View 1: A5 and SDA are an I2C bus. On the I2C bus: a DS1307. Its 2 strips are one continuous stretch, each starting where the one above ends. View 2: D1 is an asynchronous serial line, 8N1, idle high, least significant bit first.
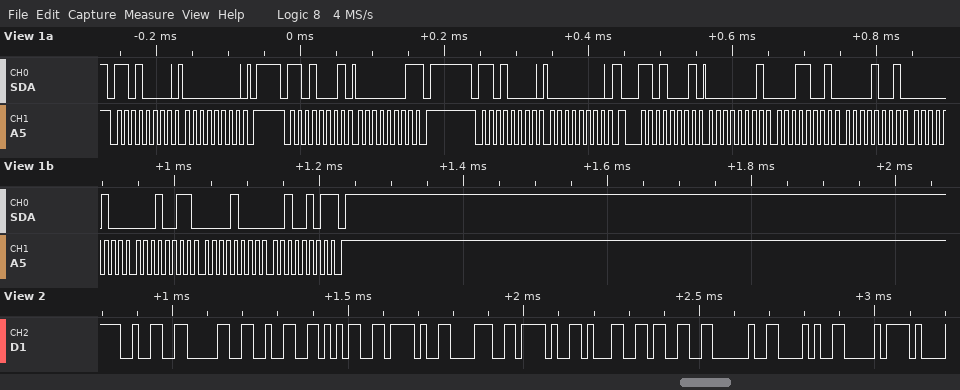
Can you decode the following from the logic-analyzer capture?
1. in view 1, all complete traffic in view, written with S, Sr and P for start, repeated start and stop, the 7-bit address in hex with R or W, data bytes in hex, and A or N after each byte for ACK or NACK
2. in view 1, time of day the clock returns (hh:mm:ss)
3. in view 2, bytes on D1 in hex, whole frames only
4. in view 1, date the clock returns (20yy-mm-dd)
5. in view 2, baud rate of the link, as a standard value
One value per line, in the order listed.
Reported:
S 68W A 00 A P S 68R A 01 N P S 68W A 00 A Sr 68R A 01 A 19 A 09 A 04 A 13 A 08 A 25 N P
09:19:01
32 30 32 35 2F 38 2F 31 33 20 28 D0
2025-08-13
57600 baud
